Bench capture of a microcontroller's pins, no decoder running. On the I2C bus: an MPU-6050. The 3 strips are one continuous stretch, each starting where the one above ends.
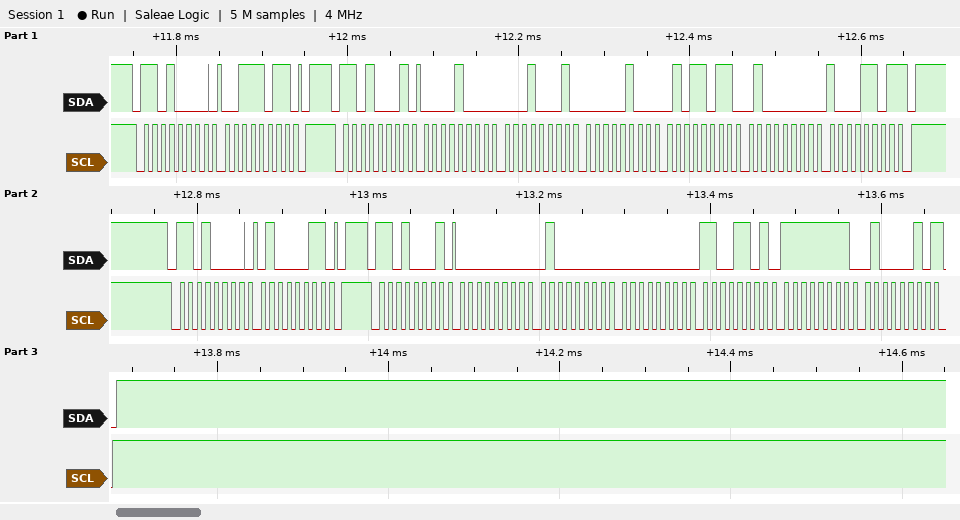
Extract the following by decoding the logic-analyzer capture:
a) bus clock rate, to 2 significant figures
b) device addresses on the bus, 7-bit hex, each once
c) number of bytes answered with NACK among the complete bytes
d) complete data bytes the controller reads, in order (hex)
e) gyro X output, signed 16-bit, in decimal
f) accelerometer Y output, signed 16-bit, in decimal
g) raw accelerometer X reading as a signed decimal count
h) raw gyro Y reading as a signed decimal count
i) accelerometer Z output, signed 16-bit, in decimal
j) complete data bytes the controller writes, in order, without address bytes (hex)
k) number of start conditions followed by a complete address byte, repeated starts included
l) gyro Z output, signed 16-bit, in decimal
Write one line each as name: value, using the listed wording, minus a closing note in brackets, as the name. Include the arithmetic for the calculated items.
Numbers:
bus clock rate, to 2 significant figures: 100 kHz
device addresses on the bus, 7-bit hex, each once: 0x68
number of bytes answered with NACK among the complete bytes: 2
complete data bytes the controller reads, in order: 08 11 04 5B 40 8D 00 40 00 CD FF 42
gyro X output, signed 16-bit, in decimal: 0x0040 = 64
accelerometer Y output, signed 16-bit, in decimal: 0x045B = 1115
raw accelerometer X reading as a signed decimal count: 0x0811 = 2065
raw gyro Y reading as a signed decimal count: 0x00CD = 205
accelerometer Z output, signed 16-bit, in decimal: 0x408D = 16525
complete data bytes the controller writes, in order, without address bytes: 3B 43
number of start conditions followed by a complete address byte, repeated starts included: 4
gyro Z output, signed 16-bit, in decimal: 0xFF42 = -190
